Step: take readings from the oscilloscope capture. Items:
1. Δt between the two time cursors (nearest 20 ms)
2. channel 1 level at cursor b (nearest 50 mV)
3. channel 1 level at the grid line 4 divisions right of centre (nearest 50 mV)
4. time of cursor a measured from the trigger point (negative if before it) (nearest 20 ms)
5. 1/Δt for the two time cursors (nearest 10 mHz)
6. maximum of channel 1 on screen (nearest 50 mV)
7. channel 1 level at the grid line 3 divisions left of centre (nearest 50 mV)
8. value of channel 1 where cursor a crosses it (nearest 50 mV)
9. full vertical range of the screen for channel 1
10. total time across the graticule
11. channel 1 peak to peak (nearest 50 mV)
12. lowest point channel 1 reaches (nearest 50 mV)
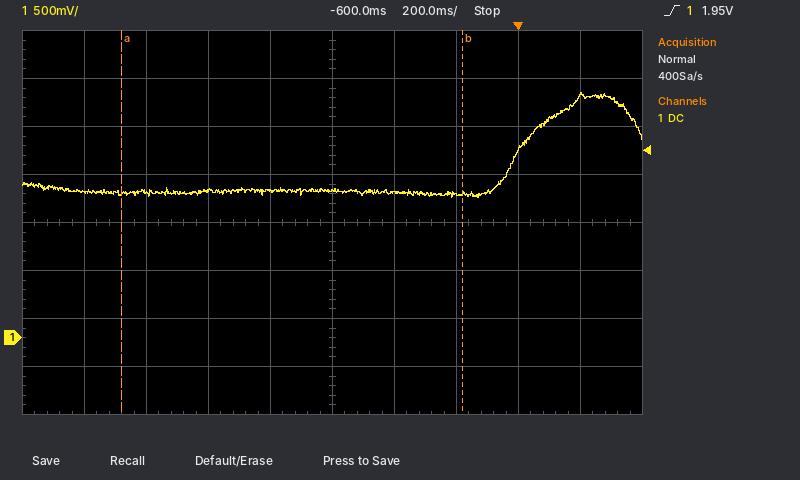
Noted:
1.10 s
1.50 V
2.50 V
-1.28 s
910 mHz
2.55 V
1.50 V
1.50 V
4 V
2 s
1.10 V
1.45 V
